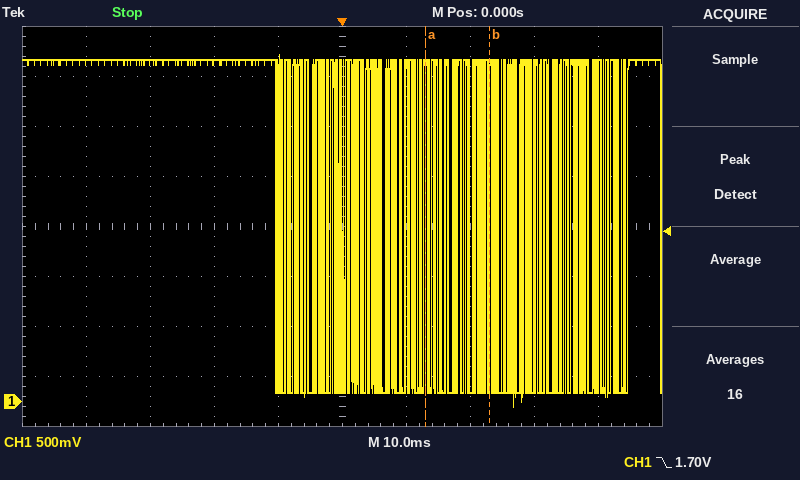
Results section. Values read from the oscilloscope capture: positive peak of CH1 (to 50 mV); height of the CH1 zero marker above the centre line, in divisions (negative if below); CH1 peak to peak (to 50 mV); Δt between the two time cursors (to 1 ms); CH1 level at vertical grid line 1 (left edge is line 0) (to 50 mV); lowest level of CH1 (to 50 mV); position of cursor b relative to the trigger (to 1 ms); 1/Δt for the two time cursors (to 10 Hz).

3.45 V
-3.5 div
3.50 V
10 ms
3.40 V
-50 mV
+23 ms
100 Hz
